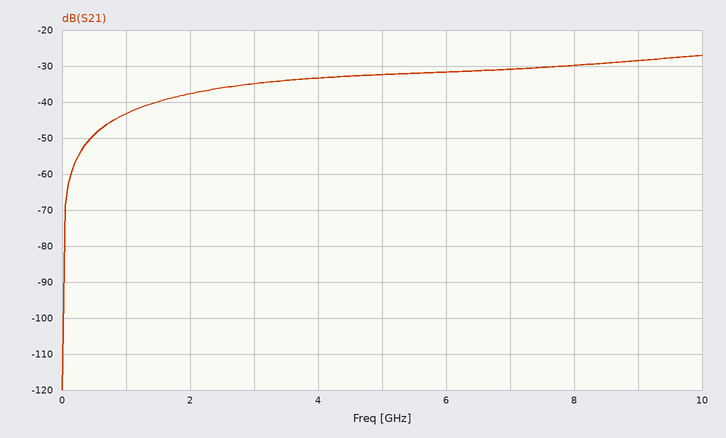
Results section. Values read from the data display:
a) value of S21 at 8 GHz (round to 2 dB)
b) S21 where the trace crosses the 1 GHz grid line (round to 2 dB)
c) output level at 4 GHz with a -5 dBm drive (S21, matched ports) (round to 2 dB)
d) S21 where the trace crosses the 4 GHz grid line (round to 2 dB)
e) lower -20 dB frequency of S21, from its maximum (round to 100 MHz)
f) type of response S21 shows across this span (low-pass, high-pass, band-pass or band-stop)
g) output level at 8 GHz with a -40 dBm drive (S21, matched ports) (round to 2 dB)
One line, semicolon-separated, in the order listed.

-30 dB; -44 dB; -38 dBm; -34 dB; 600 MHz; high-pass; -70 dBm
